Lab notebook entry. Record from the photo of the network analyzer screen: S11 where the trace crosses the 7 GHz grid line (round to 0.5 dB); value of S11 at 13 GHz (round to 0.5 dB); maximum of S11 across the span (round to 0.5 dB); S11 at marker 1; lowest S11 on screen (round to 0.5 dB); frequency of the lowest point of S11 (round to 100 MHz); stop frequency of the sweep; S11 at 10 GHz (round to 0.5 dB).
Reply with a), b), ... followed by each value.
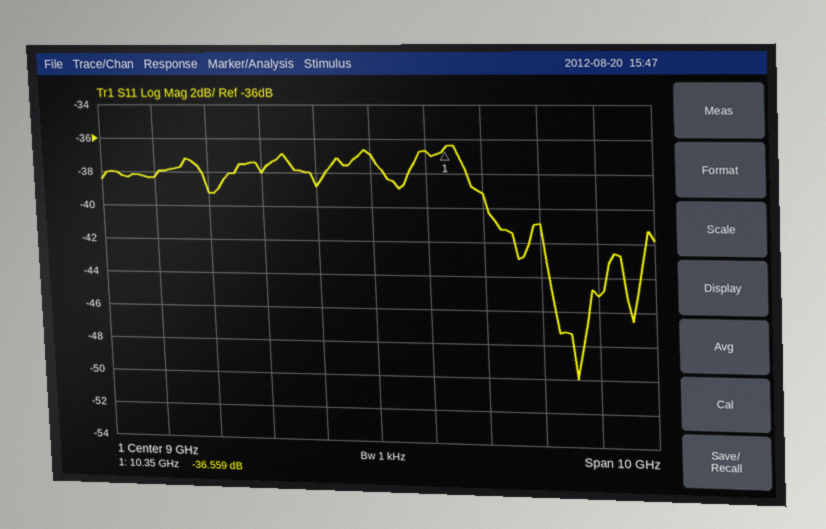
a) -38.0 dB
b) -45.0 dB
c) -36.5 dB
d) -36.559 dB
e) -50.0 dB
f) 12.6 GHz
g) 14 GHz
h) -36.5 dB
